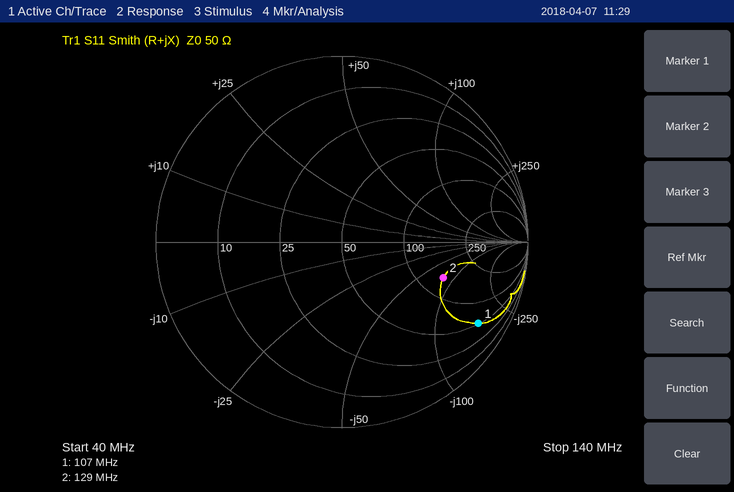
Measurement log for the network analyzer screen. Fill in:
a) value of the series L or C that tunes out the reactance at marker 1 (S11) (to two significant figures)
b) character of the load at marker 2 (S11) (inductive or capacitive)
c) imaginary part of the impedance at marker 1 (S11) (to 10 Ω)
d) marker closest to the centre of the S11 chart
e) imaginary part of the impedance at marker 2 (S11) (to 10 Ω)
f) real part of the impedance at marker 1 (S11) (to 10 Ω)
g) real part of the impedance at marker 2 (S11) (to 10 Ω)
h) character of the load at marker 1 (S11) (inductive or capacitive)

250 nH
capacitive
-170 Ω
marker 2
-80 Ω
50 Ω
140 Ω
capacitive
